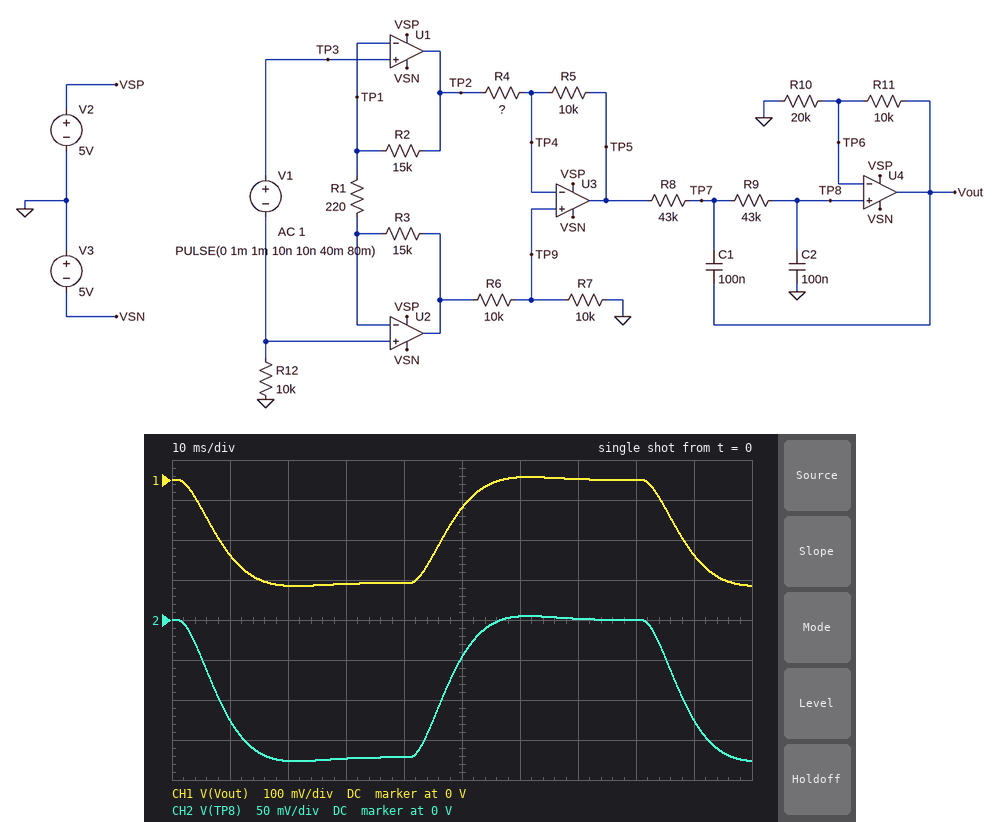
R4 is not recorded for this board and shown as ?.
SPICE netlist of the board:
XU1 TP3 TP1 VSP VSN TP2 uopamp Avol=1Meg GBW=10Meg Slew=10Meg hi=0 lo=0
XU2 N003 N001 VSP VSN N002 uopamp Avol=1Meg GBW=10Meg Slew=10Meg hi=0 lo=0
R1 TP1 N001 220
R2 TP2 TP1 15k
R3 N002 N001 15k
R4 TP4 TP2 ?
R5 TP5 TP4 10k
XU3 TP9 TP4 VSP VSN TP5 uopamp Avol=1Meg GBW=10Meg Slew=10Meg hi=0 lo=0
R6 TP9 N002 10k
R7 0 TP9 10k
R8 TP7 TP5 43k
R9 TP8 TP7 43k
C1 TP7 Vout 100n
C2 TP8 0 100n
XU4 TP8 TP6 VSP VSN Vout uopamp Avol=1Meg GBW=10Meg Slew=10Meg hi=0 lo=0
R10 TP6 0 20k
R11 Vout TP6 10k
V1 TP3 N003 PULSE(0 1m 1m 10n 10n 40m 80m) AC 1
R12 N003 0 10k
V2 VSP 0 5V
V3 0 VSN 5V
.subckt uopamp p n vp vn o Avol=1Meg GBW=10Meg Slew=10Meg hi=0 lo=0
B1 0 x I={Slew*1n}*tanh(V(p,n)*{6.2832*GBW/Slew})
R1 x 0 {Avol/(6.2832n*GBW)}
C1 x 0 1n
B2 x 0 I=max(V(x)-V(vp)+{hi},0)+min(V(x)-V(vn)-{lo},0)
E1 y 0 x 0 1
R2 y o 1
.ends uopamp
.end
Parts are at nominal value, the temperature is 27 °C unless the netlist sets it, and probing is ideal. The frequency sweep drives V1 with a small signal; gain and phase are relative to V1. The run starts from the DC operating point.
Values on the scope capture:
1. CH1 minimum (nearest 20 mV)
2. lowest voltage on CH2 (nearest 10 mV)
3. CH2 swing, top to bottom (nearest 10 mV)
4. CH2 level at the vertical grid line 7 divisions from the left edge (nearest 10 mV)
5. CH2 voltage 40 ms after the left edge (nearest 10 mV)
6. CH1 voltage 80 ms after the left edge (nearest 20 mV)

-260 mV
-180 mV
180 mV
0 V
-170 mV
0 V
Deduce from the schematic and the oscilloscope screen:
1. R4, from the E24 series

7.5 kΩ
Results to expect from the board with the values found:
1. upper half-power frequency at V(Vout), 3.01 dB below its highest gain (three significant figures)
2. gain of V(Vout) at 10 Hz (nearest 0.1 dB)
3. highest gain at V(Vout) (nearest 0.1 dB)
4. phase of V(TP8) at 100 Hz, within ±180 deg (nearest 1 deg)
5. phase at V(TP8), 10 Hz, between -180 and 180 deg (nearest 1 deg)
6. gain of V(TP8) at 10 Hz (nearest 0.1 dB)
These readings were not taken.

34.8 Hz
48.1 dB
48.2 dB
33 deg
156 deg
44.6 dB
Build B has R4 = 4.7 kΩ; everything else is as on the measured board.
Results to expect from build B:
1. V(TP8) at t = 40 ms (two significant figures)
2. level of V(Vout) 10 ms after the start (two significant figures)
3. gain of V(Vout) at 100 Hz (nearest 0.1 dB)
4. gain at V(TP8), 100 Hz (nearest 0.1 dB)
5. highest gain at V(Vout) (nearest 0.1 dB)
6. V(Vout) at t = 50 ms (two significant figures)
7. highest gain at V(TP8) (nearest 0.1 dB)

-250 mV
-280 mV
34.1 dB
30.6 dB
51.6 dB
-100 mV
48.1 dB
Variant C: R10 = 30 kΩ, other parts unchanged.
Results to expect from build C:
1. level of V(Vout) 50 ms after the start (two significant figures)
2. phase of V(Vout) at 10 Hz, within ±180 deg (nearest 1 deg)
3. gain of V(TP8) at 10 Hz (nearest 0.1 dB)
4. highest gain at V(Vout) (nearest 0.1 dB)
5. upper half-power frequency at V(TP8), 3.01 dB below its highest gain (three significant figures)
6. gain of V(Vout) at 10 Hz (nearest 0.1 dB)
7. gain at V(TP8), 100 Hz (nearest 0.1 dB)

-71 mV
154 deg
44.4 dB
47.2 dB
30.6 Hz
46.9 dB
26.9 dB
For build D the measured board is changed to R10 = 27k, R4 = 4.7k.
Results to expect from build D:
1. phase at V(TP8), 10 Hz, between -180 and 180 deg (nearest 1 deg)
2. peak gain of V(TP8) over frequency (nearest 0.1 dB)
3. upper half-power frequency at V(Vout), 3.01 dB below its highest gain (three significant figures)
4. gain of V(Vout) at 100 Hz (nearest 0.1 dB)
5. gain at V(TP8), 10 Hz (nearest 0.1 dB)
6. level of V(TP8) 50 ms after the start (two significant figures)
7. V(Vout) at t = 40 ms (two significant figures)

155 deg
48.1 dB
31.5 Hz
33.1 dB
47.9 dB
-77 mV
-350 mV
